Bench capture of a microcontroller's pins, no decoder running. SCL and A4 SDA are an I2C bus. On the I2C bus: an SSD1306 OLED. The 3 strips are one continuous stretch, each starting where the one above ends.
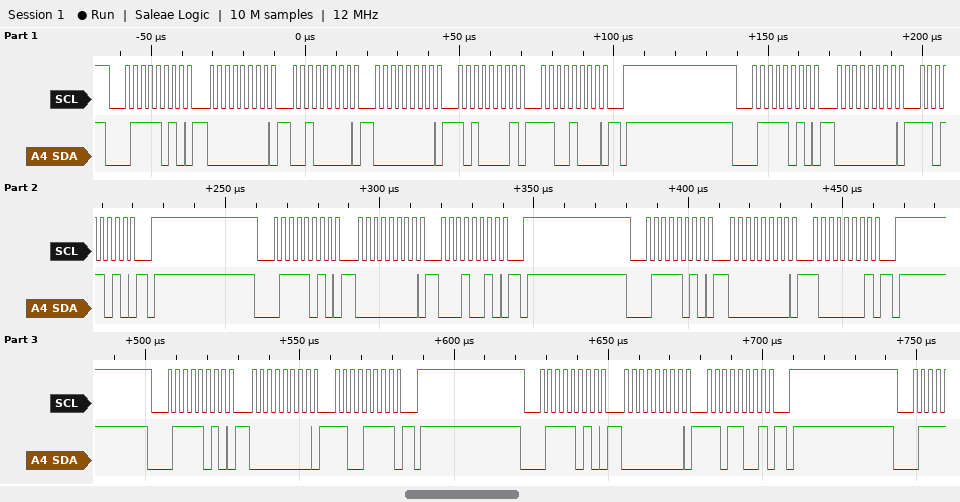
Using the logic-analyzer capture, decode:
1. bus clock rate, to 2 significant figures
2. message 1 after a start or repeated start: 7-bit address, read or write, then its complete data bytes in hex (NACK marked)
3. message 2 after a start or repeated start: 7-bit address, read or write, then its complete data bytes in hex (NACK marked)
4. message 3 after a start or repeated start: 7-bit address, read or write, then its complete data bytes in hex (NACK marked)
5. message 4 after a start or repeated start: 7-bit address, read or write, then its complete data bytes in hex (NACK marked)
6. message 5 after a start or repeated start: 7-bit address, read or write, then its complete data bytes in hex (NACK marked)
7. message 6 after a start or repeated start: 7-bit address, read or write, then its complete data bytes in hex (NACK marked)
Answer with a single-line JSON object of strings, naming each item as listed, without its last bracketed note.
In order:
{"bus clock rate, to 2 significant figures": "400 kHz", "message 1 after a start or repeated start: 7-bit address, read or write, then its complete data bytes in hex": "0x3D write: 00 20 00 A1 C8", "message 2 after a start or repeated start: 7-bit address, read or write, then its complete data bytes in hex": "0x3D write: 00 DA", "message 3 after a start or repeated start: 7-bit address, read or write, then its complete data bytes in hex": "0x3D write: 00 12", "message 4 after a start or repeated start: 7-bit address, read or write, then its complete data bytes in hex": "0x3D write: 00 81", "message 5 after a start or repeated start: 7-bit address, read or write, then its complete data bytes in hex": "0x3D write: 00 CF", "message 6 after a start or repeated start: 7-bit address, read or write, then its complete data bytes in hex": "0x3D write: 00 D9"}
